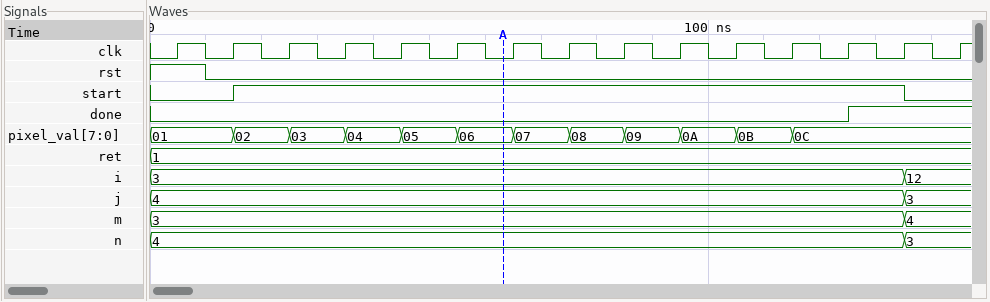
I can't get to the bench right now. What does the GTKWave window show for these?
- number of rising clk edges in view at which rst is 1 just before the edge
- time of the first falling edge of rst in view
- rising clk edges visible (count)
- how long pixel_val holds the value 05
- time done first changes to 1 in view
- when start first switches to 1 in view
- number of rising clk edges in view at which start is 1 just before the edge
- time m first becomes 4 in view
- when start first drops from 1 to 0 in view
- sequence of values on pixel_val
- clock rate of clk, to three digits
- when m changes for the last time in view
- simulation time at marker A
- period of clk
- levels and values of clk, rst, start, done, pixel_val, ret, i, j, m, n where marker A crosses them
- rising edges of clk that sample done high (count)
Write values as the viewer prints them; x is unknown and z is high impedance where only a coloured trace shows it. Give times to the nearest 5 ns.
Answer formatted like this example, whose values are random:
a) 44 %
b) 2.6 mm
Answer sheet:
a) 1
b) 10 ns
c) 15
d) 10 ns
e) 125 ns
f) 15 ns
g) 12
h) 135 ns
i) 135 ns
j) 01, 02, 03, 04, 05, 06, 07, 08, 09, 0A, 0B, 0C
k) 100 MHz
l) 135 ns
m) 65 ns
n) 10 ns
o) clk=0, rst=0, start=1, done=0, pixel_val=06, ret=1, i=3, j=4, m=3, n=4
p) 2
